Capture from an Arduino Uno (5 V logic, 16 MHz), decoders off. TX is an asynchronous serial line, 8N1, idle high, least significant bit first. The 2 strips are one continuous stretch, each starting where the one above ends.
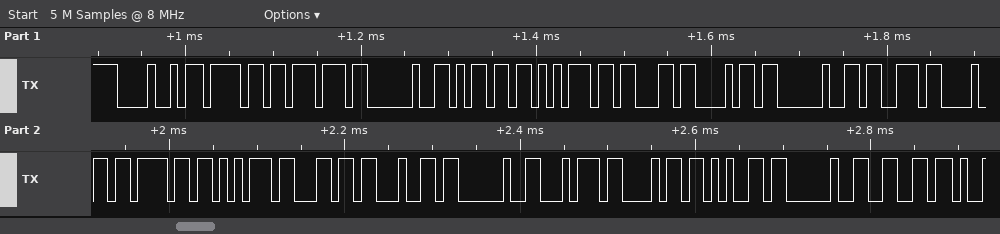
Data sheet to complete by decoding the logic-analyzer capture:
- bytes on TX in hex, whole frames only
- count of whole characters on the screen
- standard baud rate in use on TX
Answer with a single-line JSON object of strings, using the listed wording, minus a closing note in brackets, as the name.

{"bytes on TX in hex, whole frames only": "48 6F 77 20 6D 75 63 68 20 73 68 6F 75 6C 64 20 74 68 65 20 66", "count of whole characters on the screen": "21", "standard baud rate in use on TX": "115200 baud"}
